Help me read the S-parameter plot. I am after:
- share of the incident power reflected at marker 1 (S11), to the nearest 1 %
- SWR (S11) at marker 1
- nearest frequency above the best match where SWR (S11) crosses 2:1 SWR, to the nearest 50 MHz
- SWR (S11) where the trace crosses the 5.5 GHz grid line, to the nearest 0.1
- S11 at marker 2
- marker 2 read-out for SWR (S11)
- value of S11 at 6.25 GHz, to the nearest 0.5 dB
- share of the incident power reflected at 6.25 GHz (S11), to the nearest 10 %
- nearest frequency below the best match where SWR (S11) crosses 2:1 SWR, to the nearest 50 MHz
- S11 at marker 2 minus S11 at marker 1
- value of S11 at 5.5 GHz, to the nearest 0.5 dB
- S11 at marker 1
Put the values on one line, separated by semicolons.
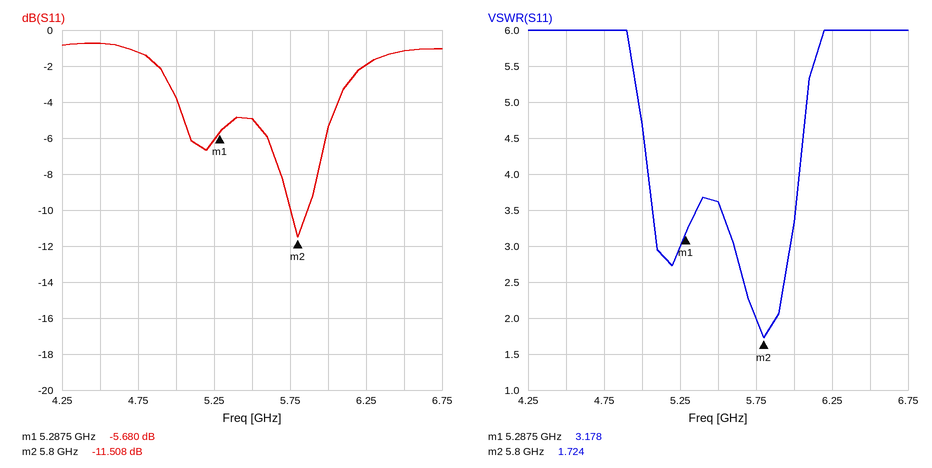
27 %; 3.178; 5.90 GHz; 3.6; -11.508 dB; 1.724; -2.0 dB; 60 %; 5.75 GHz; -5.828 dB; -5.0 dB; -5.680 dB
